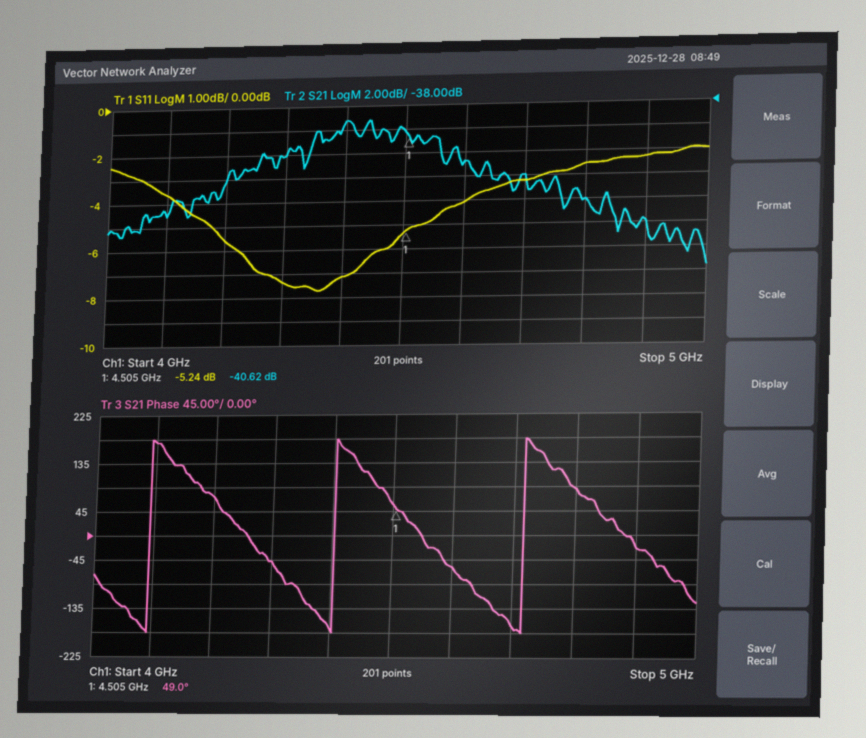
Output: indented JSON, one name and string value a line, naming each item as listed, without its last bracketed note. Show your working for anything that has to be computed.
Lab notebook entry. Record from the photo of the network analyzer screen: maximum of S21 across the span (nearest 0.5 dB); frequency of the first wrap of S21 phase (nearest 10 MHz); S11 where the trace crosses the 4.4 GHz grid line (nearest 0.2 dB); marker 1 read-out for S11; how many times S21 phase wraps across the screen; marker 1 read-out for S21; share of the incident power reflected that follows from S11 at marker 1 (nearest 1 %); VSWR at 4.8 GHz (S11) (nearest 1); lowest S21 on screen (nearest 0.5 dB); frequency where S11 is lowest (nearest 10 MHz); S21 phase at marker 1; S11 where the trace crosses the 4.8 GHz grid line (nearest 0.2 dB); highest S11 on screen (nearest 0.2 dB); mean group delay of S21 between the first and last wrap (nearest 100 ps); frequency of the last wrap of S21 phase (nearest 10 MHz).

{
  "maximum of S21 across the span": "-39.0 dB",
  "frequency of the first wrap of S21 phase": "4.09 GHz",
  "S11 where the trace crosses the 4.4 GHz grid line": "-7.2 dB",
  "marker 1 read-out for S11": "-5.24 dB",
  "how many times S21 phase wraps across the screen": "3",
  "marker 1 read-out for S21": "-40.62 dB",
  "share of the incident power reflected that follows from S11 at marker 1": "10^(-5.24/10) ≈ 30 %",
  "VSWR at 4.8 GHz (S11)": "|Γ| = 10^(-2.6/20) = 0.7413; VSWR = (1 + 0.7413)/(1 − 0.7413) ≈ 7",
  "lowest S21 on screen": "-51.5 dB",
  "frequency where S11 is lowest": "4.36 GHz",
  "S21 phase at marker 1": "49.0°",
  "S11 where the trace crosses the 4.8 GHz grid line": "-2.6 dB",
  "highest S11 on screen": "-2.0 dB",
  "mean group delay of S21 between the first and last wrap": "2 cycles / (4.72 GHz − 4.09 GHz) ≈ 3.2 ns",
  "frequency of the last wrap of S21 phase": "4.72 GHz"
}
